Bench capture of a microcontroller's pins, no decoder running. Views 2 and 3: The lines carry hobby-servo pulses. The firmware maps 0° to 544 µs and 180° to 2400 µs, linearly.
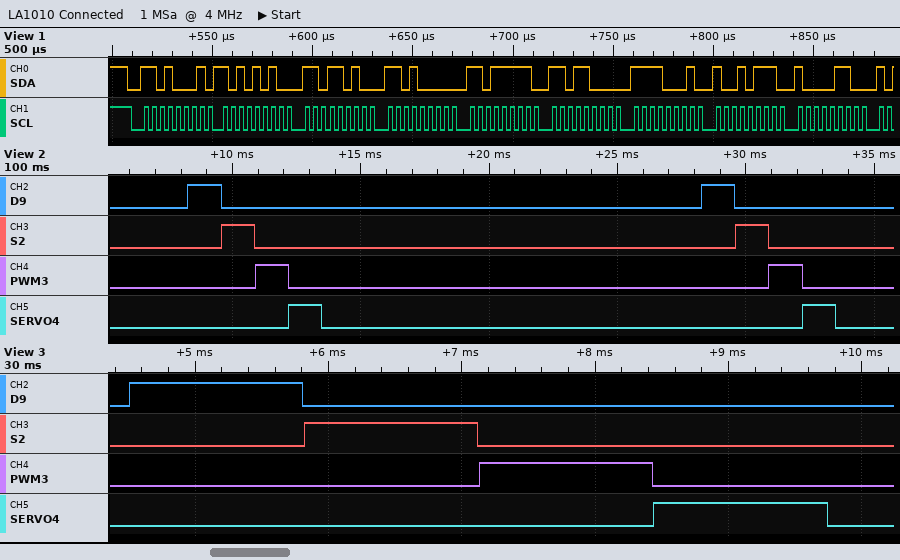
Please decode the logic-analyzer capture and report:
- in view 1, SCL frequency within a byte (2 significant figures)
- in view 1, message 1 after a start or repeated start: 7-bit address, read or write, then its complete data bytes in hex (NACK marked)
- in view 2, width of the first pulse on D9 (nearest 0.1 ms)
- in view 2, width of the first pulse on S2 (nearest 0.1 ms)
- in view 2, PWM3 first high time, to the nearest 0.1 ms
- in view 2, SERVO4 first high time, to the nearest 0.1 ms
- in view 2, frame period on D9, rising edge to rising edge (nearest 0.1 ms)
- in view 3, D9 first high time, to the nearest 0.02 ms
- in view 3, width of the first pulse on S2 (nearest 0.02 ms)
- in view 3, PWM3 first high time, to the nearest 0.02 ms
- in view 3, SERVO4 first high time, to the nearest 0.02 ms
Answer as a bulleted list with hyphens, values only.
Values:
- 250 kHz
- 0x68 read: AA DA D0 DF D8 F1 97 86
- 1.3 ms
- 1.3 ms
- 1.3 ms
- 1.3 ms
- 20.0 ms
- 1.30 ms
- 1.30 ms
- 1.30 ms
- 1.30 ms
